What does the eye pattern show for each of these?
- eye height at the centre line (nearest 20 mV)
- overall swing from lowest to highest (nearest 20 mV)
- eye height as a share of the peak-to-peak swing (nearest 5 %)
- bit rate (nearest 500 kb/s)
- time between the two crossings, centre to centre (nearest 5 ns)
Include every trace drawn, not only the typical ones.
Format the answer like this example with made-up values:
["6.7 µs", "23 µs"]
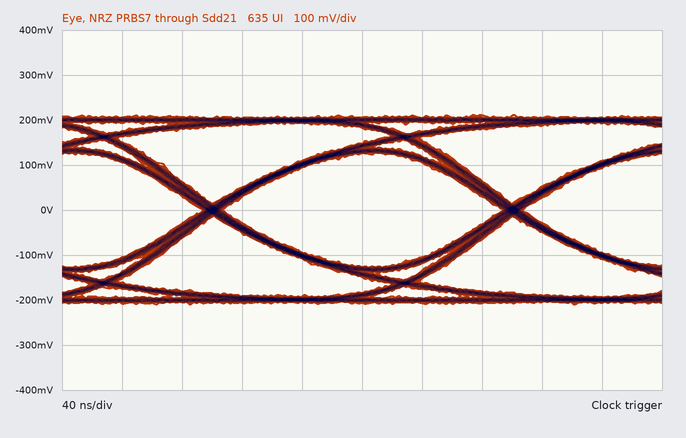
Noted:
["260 mV", "420 mV", "60 %", "5.0 Mb/s", "200 ns"]
